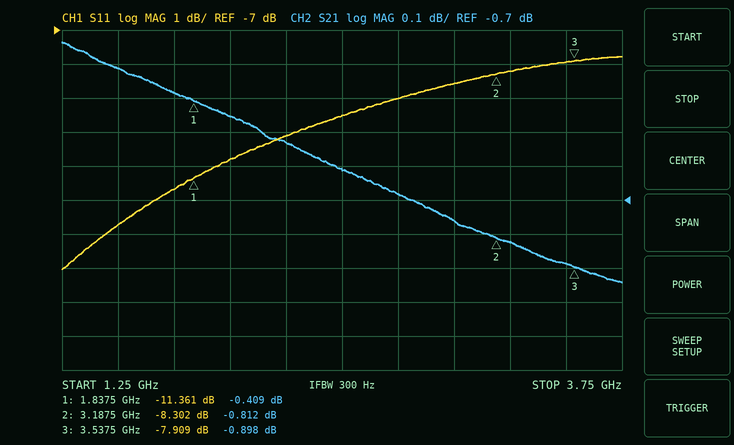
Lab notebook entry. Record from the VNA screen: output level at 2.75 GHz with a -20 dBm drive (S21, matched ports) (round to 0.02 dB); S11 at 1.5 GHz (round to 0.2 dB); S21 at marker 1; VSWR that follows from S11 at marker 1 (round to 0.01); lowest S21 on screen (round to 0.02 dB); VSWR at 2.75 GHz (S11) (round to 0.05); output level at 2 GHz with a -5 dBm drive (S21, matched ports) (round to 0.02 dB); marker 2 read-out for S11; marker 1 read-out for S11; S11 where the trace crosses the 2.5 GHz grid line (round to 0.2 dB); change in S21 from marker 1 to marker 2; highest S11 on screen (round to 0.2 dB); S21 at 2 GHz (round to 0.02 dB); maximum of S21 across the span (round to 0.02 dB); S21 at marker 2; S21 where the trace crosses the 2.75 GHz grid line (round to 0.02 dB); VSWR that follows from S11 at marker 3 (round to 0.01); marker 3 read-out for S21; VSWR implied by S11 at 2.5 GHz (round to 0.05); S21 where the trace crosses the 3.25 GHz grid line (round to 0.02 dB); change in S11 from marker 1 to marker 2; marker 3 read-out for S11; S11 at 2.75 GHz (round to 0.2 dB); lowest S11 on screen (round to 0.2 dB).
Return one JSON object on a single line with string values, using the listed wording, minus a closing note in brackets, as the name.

{"output level at 2.75 GHz with a -20 dBm drive (S21, matched ports)": "-20.68 dBm", "S11 at 1.5 GHz": "-12.8 dB", "S21 at marker 1": "-0.409 dB", "VSWR that follows from S11 at marker 1": "1.74", "lowest S21 on screen": "-0.94 dB", "VSWR at 2.75 GHz (S11)": "2.10", "output level at 2 GHz with a -5 dBm drive (S21, matched ports)": "-5.46 dBm", "marker 2 read-out for S11": "-8.302 dB", "marker 1 read-out for S11": "-11.361 dB", "S11 where the trace crosses the 2.5 GHz grid line": "-9.6 dB", "change in S21 from marker 1 to marker 2": "-0.403 dB", "highest S11 on screen": "-7.8 dB", "S21 at 2 GHz": "-0.46 dB", "maximum of S21 across the span": "-0.24 dB", "S21 at marker 2": "-0.812 dB", "S21 where the trace crosses the 2.75 GHz grid line": "-0.68 dB", "VSWR that follows from S11 at marker 3": "2.35", "marker 3 read-out for S21": "-0.898 dB", "VSWR implied by S11 at 2.5 GHz": "2.00", "S21 where the trace crosses the 3.25 GHz grid line": "-0.82 dB", "change in S11 from marker 1 to marker 2": "3.059 dB", "marker 3 read-out for S11": "-7.909 dB", "S11 at 2.75 GHz": "-9.0 dB", "lowest S11 on screen": "-14.0 dB"}
